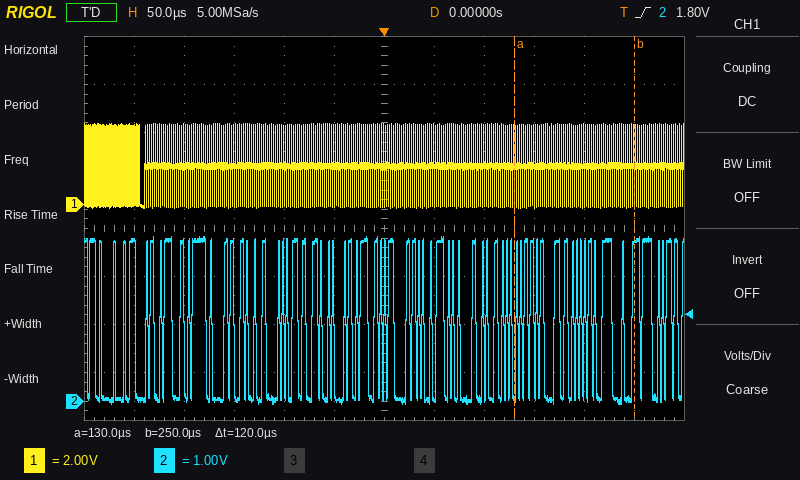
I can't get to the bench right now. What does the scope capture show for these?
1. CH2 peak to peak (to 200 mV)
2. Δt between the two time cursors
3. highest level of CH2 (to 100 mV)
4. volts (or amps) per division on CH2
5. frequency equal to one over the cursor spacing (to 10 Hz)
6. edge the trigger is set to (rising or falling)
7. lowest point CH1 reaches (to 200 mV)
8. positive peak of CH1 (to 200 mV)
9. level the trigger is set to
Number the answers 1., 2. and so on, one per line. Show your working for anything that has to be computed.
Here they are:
1. 3.4 V
2. 120 µs
3. 3.4 V
4. 1 V
5. 1 / 120 µs ≈ 8.33 kHz
6. rising
7. -200 mV
8. 3.4 V
9. 1.80 V
